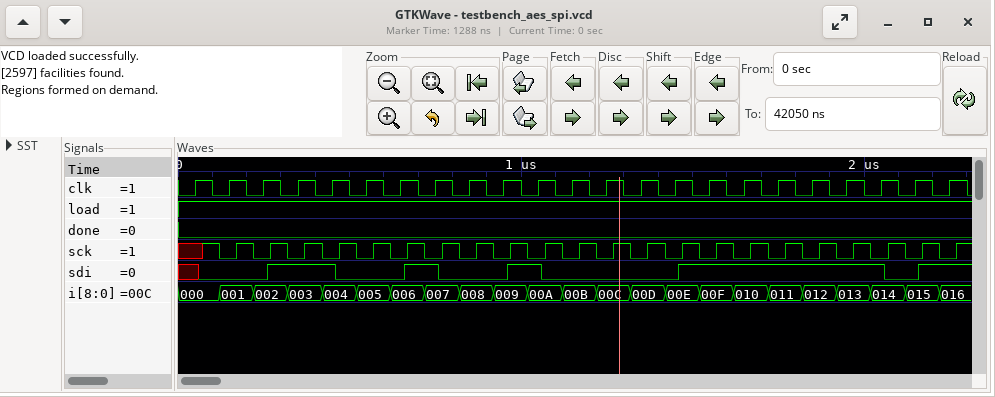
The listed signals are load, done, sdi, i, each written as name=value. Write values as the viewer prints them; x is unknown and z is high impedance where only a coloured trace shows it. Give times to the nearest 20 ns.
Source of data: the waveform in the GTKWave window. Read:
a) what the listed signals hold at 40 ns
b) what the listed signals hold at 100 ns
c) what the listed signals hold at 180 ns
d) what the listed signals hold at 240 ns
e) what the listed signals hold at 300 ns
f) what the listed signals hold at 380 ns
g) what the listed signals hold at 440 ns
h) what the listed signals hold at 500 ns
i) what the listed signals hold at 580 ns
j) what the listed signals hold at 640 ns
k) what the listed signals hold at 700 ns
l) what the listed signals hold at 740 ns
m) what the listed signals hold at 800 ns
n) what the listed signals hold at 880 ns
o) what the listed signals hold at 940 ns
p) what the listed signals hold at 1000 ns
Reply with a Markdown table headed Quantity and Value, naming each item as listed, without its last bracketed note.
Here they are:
| Quantity | Value |
|---|---|
| what the listed signals hold at 40 ns | load=1, done=0, sdi=x, i=000 |
| what the listed signals hold at 100 ns | load=1, done=0, sdi=0, i=000 |
| what the listed signals hold at 180 ns | load=1, done=0, sdi=0, i=001 |
| what the listed signals hold at 240 ns | load=1, done=0, sdi=0, i=002 |
| what the listed signals hold at 300 ns | load=1, done=0, sdi=1, i=002 |
| what the listed signals hold at 380 ns | load=1, done=0, sdi=1, i=003 |
| what the listed signals hold at 440 ns | load=1, done=0, sdi=1, i=004 |
| what the listed signals hold at 500 ns | load=1, done=0, sdi=0, i=004 |
| what the listed signals hold at 580 ns | load=1, done=0, sdi=0, i=005 |
| what the listed signals hold at 640 ns | load=1, done=0, sdi=0, i=006 |
| what the listed signals hold at 700 ns | load=1, done=0, sdi=1, i=006 |
| what the listed signals hold at 740 ns | load=1, done=0, sdi=1, i=007 |
| what the listed signals hold at 800 ns | load=1, done=0, sdi=0, i=007 |
| what the listed signals hold at 880 ns | load=1, done=0, sdi=0, i=008 |
| what the listed signals hold at 940 ns | load=1, done=0, sdi=0, i=009 |
| what the listed signals hold at 1000 ns | load=1, done=0, sdi=1, i=009 |
